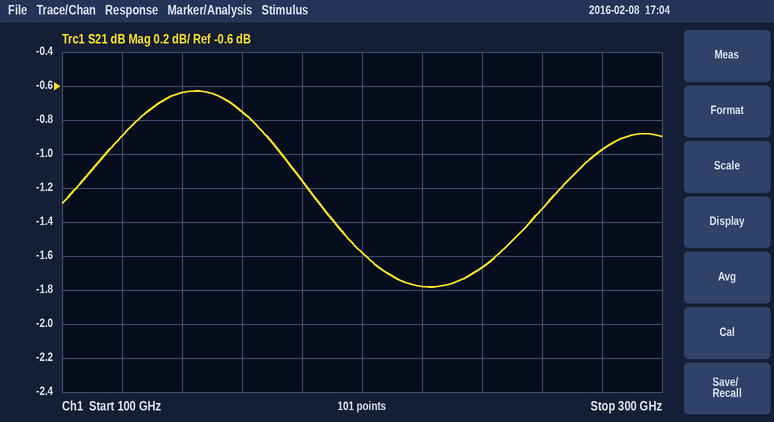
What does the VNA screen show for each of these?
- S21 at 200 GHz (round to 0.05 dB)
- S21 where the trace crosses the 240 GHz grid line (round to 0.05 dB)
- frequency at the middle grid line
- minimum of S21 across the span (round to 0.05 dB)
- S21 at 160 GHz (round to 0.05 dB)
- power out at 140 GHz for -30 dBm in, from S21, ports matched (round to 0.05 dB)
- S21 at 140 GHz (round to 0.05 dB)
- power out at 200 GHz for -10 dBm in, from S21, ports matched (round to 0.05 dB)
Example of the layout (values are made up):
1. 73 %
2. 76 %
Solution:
1. -1.60 dB
2. -1.65 dB
3. 200 GHz
4. -1.80 dB
5. -0.75 dB
6. -30.65 dBm
7. -0.65 dB
8. -11.60 dBm
